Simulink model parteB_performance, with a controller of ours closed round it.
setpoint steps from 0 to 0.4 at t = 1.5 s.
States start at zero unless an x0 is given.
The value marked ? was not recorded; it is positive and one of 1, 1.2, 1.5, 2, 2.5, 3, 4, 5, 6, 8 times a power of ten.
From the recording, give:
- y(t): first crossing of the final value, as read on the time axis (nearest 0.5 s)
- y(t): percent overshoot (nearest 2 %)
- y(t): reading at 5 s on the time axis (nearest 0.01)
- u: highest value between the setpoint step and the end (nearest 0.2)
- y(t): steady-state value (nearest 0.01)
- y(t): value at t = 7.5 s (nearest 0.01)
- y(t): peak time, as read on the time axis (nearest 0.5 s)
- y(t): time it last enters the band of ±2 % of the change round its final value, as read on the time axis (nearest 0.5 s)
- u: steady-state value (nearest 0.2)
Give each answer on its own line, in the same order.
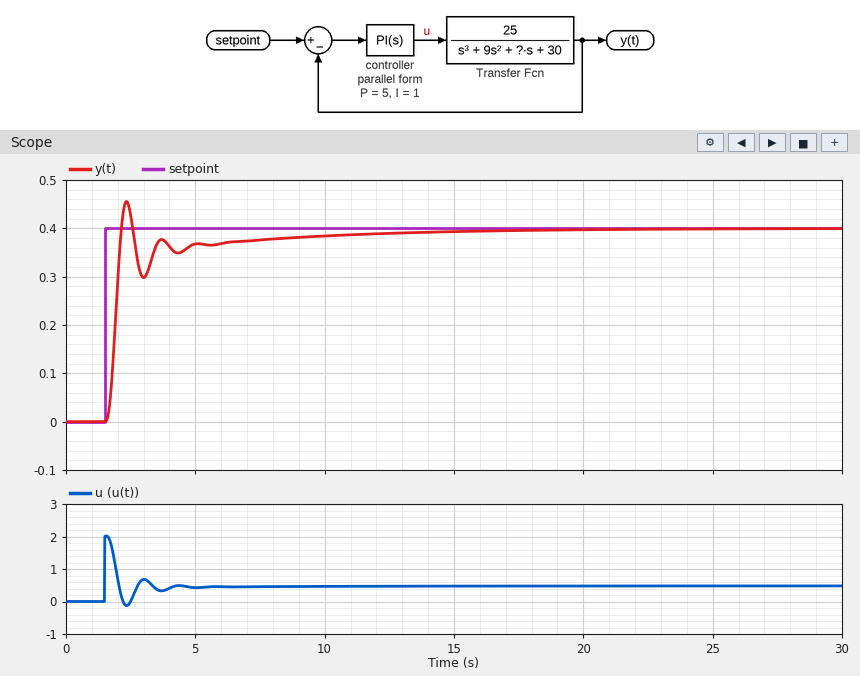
2.0 s
14 %
0.37
2.0
0.40
0.38
2.5 s
14.0 s
0.4
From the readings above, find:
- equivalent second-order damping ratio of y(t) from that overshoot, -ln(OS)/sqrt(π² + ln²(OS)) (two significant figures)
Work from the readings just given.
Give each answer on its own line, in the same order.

0.53
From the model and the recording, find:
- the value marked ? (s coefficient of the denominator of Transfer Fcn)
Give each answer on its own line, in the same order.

40
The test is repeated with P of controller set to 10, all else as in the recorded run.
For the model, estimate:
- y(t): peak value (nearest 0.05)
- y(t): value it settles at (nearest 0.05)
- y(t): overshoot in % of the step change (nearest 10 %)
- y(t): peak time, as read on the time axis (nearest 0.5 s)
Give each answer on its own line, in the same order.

0.60
0.40
50 %
2.0 s
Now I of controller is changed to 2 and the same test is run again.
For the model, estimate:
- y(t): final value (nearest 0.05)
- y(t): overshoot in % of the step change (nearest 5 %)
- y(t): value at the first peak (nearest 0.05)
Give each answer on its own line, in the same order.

0.40
20 %
0.50
